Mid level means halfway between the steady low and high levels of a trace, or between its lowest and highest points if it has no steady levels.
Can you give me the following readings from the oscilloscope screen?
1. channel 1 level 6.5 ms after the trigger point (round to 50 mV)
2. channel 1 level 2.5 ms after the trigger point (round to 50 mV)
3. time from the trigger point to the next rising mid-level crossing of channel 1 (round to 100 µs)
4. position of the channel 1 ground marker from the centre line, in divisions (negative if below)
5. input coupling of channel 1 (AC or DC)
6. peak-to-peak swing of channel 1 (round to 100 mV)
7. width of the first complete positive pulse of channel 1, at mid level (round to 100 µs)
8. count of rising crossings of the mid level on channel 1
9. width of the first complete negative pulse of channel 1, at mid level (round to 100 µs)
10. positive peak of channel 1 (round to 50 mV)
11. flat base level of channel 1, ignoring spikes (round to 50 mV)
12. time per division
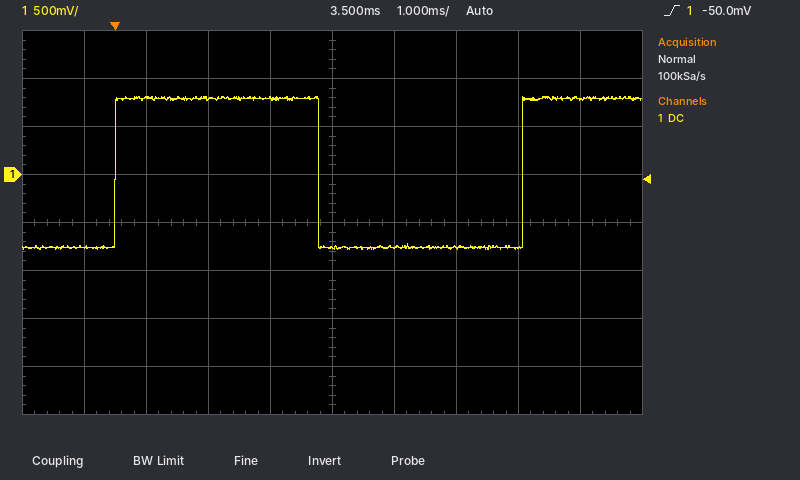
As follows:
-750 mV
800 mV
6.6 ms
+1.0 div
DC
1.60 V
3.3 ms
2
3.3 ms
800 mV
-750 mV
1 ms
